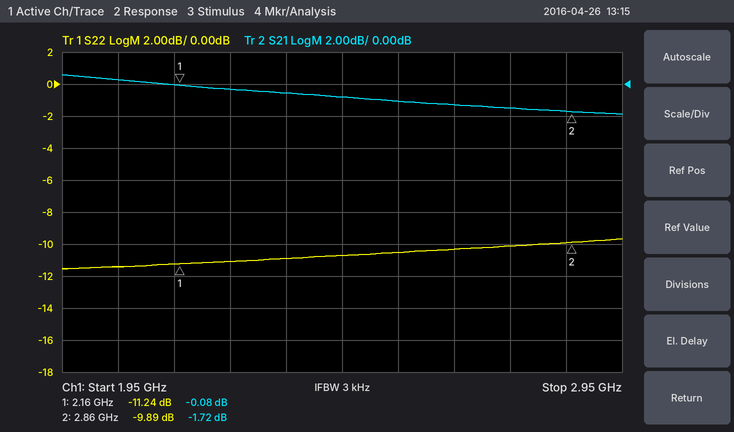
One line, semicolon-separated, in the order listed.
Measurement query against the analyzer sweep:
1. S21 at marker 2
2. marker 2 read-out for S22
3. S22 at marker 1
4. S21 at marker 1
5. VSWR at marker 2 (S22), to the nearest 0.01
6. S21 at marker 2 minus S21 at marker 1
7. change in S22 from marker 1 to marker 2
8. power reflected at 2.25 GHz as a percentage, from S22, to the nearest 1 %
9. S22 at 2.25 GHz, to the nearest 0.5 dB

-1.72 dB; -9.89 dB; -11.24 dB; -0.08 dB; 1.94; -1.64 dB; 1.35 dB; 8 %; -11.0 dB
